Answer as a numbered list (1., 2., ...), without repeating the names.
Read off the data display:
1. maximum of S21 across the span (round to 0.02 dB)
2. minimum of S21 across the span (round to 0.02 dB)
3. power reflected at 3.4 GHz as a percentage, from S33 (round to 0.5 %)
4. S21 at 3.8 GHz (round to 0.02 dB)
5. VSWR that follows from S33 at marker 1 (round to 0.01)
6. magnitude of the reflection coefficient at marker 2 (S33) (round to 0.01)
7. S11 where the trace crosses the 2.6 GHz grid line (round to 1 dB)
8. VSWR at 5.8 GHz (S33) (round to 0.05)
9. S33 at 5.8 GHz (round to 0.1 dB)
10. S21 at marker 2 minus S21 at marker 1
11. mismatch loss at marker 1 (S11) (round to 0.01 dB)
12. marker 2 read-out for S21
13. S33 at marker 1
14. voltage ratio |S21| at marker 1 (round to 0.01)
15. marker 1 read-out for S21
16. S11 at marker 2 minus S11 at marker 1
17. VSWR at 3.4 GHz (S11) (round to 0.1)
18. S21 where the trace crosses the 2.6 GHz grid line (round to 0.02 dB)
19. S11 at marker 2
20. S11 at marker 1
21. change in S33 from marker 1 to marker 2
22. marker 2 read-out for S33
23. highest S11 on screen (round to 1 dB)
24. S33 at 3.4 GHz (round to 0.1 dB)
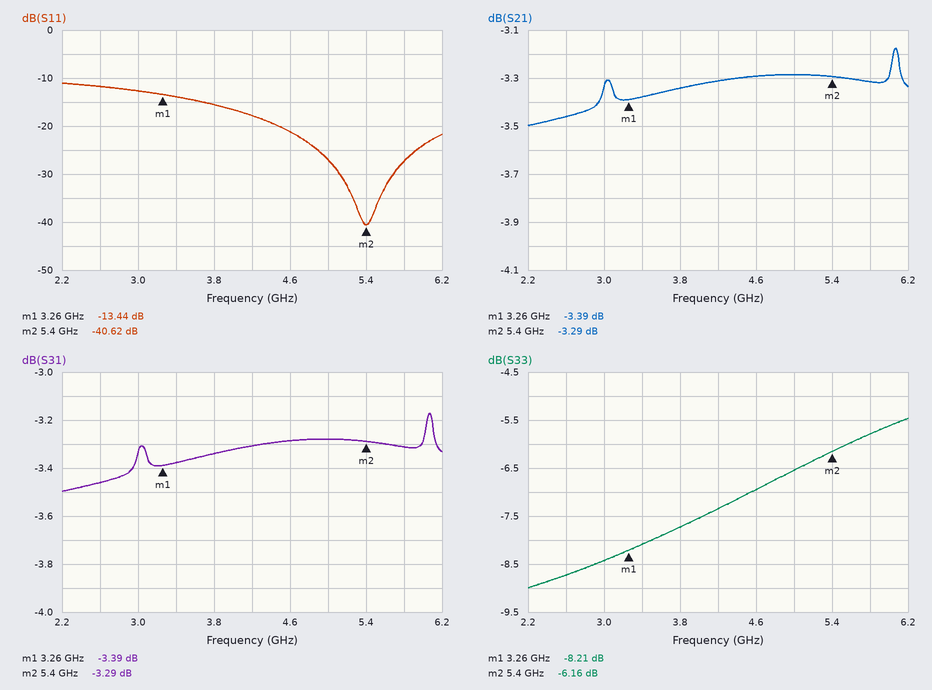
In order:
1. -3.18 dB
2. -3.50 dB
3. 15.5 %
4. -3.34 dB
5. 2.27
6. 0.49
7. -12 dB
8. 3.10
9. -5.8 dB
10. 0.10 dB
11. 0.20 dB
12. -3.29 dB
13. -8.21 dB
14. 0.68
15. -3.39 dB
16. -27.18 dB
17. 1.5
18. -3.46 dB
19. -40.62 dB
20. -13.44 dB
21. 2.05 dB
22. -6.16 dB
23. -11 dB
24. -8.1 dB
